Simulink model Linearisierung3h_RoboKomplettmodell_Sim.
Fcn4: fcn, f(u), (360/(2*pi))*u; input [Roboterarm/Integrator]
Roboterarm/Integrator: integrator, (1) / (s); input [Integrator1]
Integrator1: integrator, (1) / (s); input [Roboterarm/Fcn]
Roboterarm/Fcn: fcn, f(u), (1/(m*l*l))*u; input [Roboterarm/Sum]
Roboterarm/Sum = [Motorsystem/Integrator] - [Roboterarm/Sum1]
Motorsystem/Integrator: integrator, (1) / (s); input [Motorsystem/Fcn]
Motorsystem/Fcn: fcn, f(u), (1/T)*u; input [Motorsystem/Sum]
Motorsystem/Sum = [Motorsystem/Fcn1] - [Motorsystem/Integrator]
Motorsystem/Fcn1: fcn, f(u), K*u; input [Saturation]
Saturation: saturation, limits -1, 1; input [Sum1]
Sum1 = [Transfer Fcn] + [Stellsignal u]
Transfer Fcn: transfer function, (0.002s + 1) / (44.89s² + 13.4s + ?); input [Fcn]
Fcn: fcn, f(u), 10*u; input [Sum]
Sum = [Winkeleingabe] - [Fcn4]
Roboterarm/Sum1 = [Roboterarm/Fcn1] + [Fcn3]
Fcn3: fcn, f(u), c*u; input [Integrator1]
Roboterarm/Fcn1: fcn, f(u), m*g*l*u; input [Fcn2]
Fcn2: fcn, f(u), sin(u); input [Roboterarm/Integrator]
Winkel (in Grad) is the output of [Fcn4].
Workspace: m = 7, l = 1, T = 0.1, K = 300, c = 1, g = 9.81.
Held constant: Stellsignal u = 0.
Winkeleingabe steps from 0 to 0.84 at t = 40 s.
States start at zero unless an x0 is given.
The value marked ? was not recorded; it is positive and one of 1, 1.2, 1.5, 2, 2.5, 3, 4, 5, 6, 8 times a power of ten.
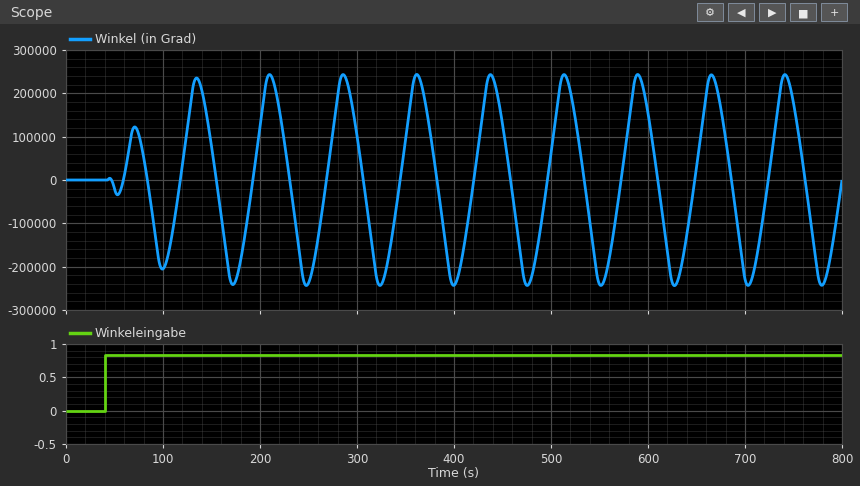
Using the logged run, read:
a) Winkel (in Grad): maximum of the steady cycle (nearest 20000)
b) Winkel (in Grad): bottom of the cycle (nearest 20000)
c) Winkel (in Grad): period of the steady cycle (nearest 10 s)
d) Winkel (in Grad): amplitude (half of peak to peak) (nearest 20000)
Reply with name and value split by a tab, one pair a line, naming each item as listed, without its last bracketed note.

Winkel (in Grad): maximum of the steady cycle	240000
Winkel (in Grad): bottom of the cycle	-240000
Winkel (in Grad): period of the steady cycle	80 s
Winkel (in Grad): amplitude (half of peak to peak)	240000
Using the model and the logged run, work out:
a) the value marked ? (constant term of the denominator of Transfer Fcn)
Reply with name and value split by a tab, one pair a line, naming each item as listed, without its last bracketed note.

the value marked ?	1
